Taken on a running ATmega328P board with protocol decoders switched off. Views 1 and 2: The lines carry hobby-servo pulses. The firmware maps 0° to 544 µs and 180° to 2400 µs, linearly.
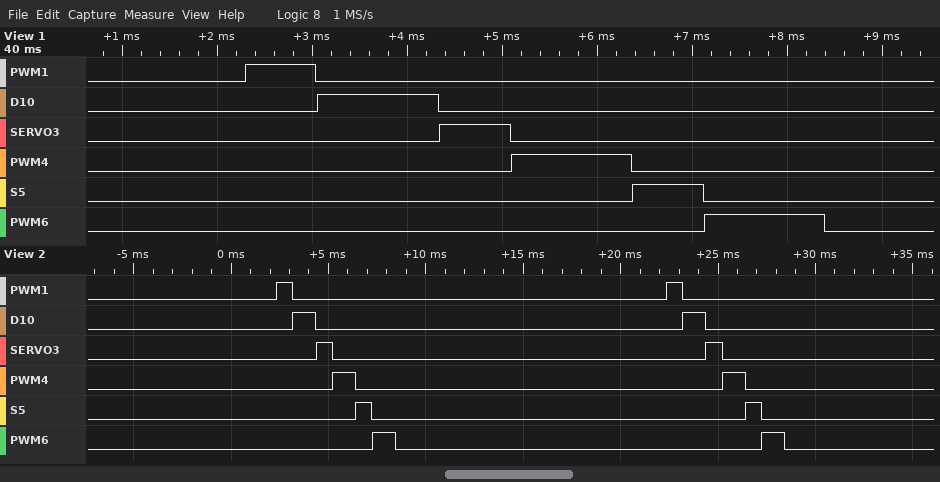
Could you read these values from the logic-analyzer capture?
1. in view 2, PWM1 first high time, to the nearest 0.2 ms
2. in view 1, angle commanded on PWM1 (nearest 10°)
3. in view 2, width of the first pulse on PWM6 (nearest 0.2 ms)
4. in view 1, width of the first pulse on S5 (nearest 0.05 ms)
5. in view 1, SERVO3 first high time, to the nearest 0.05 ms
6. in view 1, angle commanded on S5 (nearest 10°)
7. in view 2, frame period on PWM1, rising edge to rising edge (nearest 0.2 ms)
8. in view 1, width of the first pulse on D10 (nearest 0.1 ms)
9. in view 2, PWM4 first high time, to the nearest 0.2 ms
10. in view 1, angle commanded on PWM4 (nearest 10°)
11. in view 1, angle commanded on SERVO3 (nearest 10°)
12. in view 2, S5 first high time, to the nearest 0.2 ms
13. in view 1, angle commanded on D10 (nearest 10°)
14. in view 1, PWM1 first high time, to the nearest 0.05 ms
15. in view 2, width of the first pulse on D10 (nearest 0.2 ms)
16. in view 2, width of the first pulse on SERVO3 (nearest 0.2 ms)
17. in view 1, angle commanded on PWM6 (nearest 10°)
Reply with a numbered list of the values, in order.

1. 0.8 ms
2. 20°
3. 1.2 ms
4. 0.75 ms
5. 0.75 ms
6. 20°
7. 20.0 ms
8. 1.3 ms
9. 1.2 ms
10. 70°
11. 20°
12. 0.8 ms
13. 70°
14. 0.75 ms
15. 1.2 ms
16. 0.8 ms
17. 70°
